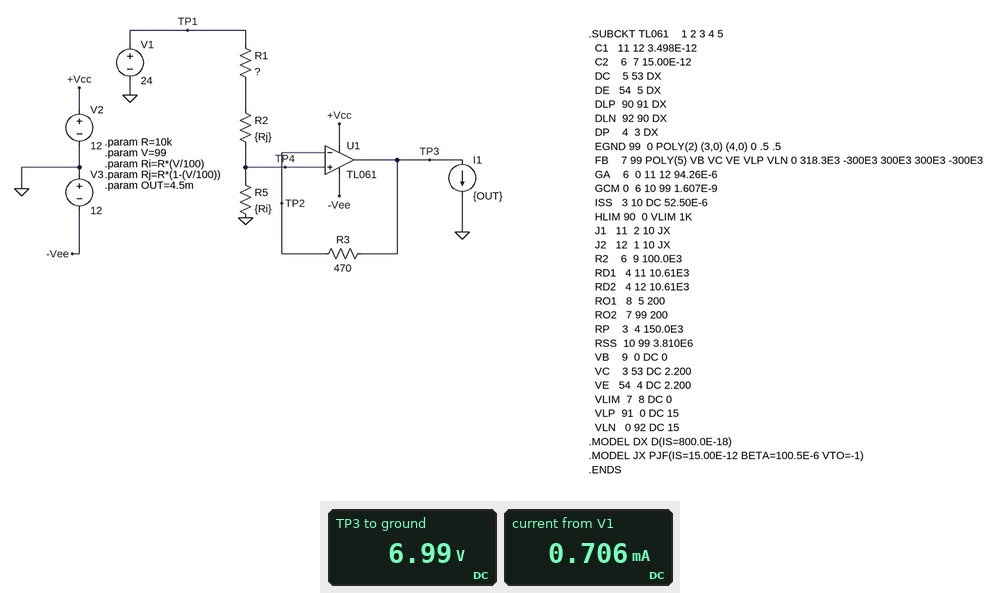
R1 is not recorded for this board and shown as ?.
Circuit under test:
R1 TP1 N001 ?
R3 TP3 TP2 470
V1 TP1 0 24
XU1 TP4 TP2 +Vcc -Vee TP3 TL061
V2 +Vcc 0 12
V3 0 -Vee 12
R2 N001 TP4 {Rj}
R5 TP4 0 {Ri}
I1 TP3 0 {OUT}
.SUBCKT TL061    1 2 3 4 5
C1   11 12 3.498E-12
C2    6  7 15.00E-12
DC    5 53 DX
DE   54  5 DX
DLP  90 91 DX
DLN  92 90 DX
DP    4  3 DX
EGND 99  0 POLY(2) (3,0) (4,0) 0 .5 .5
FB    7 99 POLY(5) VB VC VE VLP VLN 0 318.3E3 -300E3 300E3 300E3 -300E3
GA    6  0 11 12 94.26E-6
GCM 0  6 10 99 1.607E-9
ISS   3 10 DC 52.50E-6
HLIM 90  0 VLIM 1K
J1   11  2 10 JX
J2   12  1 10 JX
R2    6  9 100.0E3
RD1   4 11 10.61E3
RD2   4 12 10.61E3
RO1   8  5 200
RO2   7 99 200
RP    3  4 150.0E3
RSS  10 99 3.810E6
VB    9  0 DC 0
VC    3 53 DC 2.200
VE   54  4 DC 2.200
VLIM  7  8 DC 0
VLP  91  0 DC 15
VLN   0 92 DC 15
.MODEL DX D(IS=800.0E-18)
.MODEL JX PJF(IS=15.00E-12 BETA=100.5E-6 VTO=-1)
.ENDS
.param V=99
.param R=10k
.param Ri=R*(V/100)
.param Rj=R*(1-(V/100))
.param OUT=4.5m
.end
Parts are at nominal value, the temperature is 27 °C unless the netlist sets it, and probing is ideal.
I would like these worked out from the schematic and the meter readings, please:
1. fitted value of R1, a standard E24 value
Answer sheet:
24 kΩ
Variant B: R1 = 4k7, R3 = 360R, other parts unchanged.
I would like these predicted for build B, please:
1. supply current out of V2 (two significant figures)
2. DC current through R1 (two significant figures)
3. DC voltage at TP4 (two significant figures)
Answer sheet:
160 µA
1.6 mA
16 V
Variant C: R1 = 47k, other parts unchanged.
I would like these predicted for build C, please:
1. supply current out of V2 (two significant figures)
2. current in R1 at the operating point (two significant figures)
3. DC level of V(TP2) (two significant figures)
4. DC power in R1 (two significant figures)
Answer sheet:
210 µA
420 µA
4.2 V
8.3 mW
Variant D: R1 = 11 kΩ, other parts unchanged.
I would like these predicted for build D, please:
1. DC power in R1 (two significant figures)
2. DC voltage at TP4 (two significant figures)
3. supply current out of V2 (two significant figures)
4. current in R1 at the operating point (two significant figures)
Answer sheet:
14 mW
11 V
160 µA
1.1 mA
